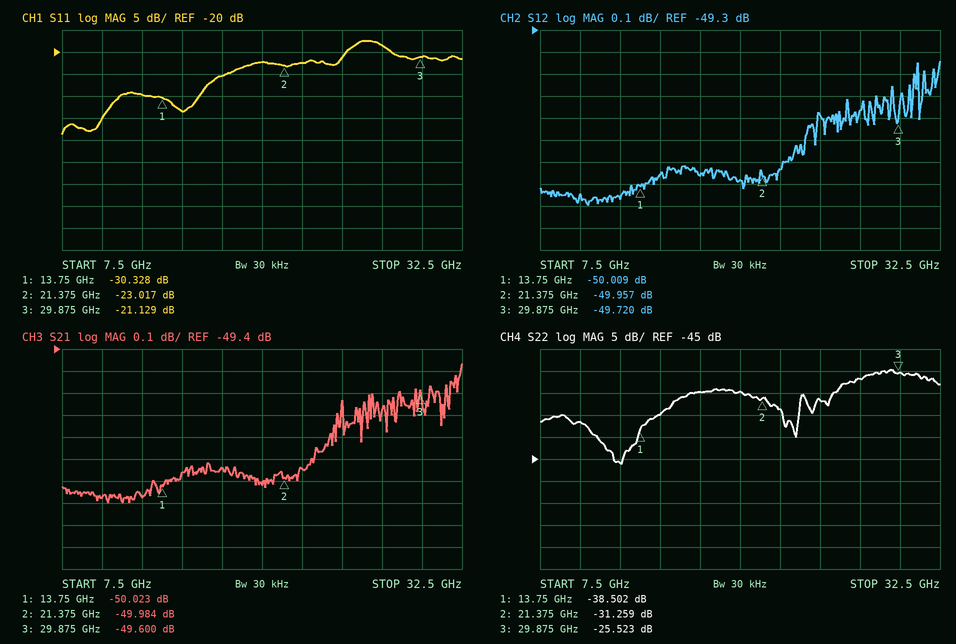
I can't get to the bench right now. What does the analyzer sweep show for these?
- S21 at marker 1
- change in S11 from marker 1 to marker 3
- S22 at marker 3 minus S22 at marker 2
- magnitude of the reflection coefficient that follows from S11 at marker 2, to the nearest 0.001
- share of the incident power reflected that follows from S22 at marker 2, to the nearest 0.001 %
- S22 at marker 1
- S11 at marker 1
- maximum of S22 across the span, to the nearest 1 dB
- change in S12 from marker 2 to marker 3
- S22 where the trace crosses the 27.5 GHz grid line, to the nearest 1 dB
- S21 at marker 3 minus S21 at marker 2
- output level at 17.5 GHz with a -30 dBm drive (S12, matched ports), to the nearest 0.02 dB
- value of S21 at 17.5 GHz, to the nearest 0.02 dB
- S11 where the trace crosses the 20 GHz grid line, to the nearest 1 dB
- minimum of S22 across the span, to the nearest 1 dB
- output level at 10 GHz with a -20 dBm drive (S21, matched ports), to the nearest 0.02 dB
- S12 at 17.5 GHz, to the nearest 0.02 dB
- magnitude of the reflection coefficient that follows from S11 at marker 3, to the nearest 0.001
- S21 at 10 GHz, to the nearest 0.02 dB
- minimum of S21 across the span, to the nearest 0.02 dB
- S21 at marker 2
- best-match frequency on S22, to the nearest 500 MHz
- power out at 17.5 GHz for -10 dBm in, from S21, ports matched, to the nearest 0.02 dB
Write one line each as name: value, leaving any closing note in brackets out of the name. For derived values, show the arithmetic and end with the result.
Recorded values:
S21 at marker 1: -50.023 dB
change in S11 from marker 1 to marker 3: -21.129 − (-30.328) = 9.199 dB
S22 at marker 3 minus S22 at marker 2: -25.523 − (-31.259) = 5.736 dB
magnitude of the reflection coefficient that follows from S11 at marker 2, to the nearest 0.001: 10^(-23.017/20) ≈ 0.071
share of the incident power reflected that follows from S22 at marker 2, to the nearest 0.001 %: 10^(-31.259/10) ≈ 0.075 %
S22 at marker 1: -38.502 dB
S11 at marker 1: -30.328 dB
maximum of S22 across the span, to the nearest 1 dB: -25 dB
change in S12 from marker 2 to marker 3: -49.72 − (-49.957) = 0.237 dB
S22 where the trace crosses the 27.5 GHz grid line, to the nearest 1 dB: -27 dB
S21 at marker 3 minus S21 at marker 2: -49.6 − (-49.984) = 0.384 dB
output level at 17.5 GHz with a -30 dBm drive (S12, matched ports), to the nearest 0.02 dB: -30 dBm + (-49.96 dB) = -79.96 dBm
value of S21 at 17.5 GHz, to the nearest 0.02 dB: -49.94 dB
S11 where the trace crosses the 20 GHz grid line, to the nearest 1 dB: -22 dB
minimum of S22 across the span, to the nearest 1 dB: -46 dB
output level at 10 GHz with a -20 dBm drive (S21, matched ports), to the nearest 0.02 dB: -20 dBm + (-50.08 dB) = -70.08 dBm
S12 at 17.5 GHz, to the nearest 0.02 dB: -49.96 dB
magnitude of the reflection coefficient that follows from S11 at marker 3, to the nearest 0.001: 10^(-21.129/20) ≈ 0.088
S21 at 10 GHz, to the nearest 0.02 dB: -50.08 dB
minimum of S21 across the span, to the nearest 0.02 dB: -50.10 dB
S21 at marker 2: -49.984 dB
best-match frequency on S22, to the nearest 500 MHz: 12.5 GHz
power out at 17.5 GHz for -10 dBm in, from S21, ports matched, to the nearest 0.02 dB: -10 dBm + (-49.94 dB) = -59.94 dBm
